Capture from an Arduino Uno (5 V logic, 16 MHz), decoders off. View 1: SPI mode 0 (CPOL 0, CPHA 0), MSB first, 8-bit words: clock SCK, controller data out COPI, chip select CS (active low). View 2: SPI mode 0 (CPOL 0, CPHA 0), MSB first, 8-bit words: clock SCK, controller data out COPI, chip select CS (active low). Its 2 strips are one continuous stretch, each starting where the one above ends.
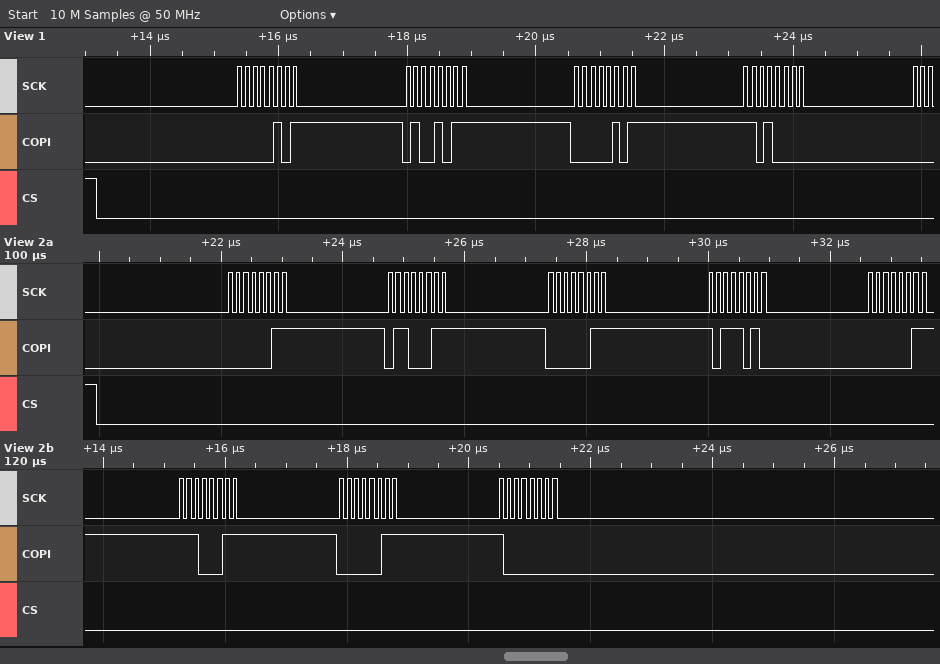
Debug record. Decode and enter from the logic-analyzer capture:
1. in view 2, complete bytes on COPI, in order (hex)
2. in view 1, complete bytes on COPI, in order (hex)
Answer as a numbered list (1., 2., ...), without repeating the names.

1. 03 63 03 BA 03 E3 03 80
2. 0x05 0x4B 0x05 0xD0
